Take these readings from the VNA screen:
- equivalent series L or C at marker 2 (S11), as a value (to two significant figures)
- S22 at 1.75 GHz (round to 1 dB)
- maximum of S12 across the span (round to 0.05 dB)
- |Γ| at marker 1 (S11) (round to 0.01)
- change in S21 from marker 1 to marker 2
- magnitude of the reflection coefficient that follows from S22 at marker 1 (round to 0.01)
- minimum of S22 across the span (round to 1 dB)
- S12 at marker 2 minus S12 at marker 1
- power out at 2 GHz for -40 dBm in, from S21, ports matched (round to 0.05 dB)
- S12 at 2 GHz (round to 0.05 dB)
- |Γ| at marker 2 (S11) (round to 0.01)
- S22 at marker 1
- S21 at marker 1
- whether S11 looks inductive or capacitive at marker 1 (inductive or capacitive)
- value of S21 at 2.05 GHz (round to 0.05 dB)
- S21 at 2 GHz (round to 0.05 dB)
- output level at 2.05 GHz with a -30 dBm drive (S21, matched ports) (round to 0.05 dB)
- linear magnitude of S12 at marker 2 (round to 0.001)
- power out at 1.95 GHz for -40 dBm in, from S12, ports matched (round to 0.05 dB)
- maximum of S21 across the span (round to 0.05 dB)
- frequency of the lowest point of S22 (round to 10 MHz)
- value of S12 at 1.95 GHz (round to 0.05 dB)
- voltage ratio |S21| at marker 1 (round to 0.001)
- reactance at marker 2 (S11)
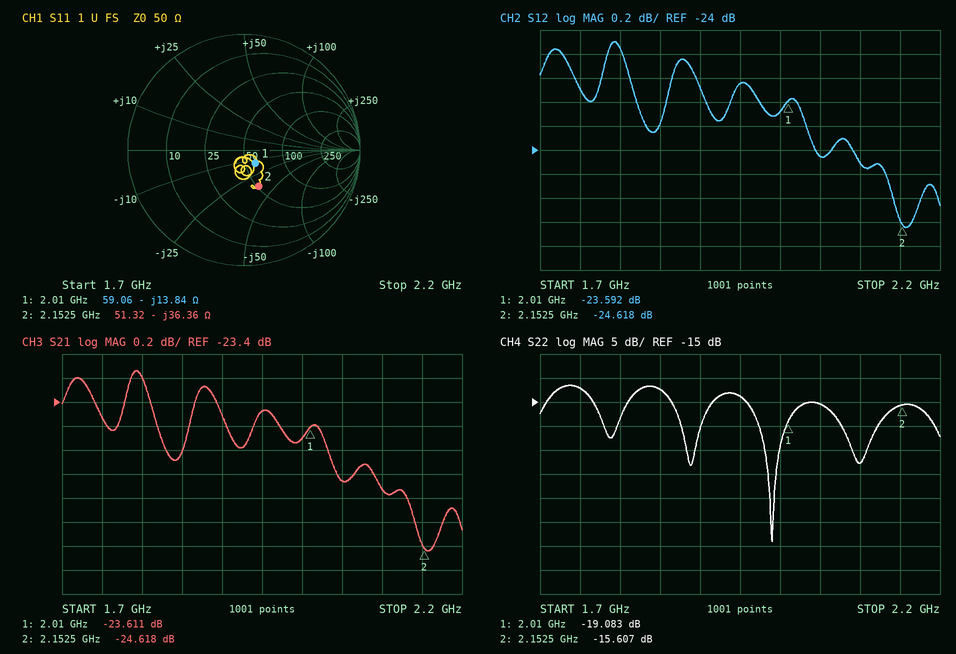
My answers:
2.0 pF
-12 dB
-23.10 dB
0.15
-1.007 dB
0.11
-44 dB
-1.026 dB
-63.70 dBm
-23.70 dB
0.34
-19.083 dB
-23.611 dB
capacitive
-24.05 dB
-23.70 dB
-54.05 dBm
0.059
-63.45 dBm
-23.15 dB
1.99 GHz
-23.45 dB
0.066
-36.36 Ω
